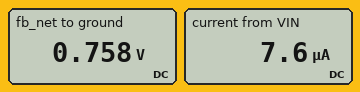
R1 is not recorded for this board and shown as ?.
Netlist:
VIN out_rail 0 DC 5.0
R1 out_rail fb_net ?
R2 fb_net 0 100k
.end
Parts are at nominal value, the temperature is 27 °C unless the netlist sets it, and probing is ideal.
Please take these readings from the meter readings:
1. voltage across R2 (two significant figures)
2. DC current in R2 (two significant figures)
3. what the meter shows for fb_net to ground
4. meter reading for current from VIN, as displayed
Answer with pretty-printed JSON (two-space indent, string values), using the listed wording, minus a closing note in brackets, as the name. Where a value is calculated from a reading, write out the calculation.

{
  "voltage across R2": "758 mV = 760 mV",
  "DC current in R2": "(758 mV) / 100 kΩ = 7.6 µA",
  "what the meter shows for fb_net to ground": "0.758 V",
  "meter reading for current from VIN, as displayed": "7.6 µA"
}
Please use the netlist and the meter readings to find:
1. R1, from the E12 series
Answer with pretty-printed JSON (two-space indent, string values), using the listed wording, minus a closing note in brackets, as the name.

{
  "R1, from the E12 series": "560 kΩ"
}
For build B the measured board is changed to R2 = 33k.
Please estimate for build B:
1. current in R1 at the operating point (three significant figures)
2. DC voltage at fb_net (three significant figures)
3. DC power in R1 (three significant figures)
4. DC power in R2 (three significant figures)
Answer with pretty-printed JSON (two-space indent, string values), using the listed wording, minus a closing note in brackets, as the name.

{
  "current in R1 at the operating point": "8.43 µA",
  "DC voltage at fb_net": "278 mV",
  "DC power in R1": "39.8 µW",
  "DC power in R2": "2.35 µW"
}
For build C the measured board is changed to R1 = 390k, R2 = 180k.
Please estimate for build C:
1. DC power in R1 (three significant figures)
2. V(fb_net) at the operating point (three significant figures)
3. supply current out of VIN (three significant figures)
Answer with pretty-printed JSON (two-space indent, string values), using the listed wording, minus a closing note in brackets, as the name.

{
  "DC power in R1": "30.0 µW",
  "V(fb_net) at the operating point": "1.58 V",
  "supply current out of VIN": "8.77 µA"
}
